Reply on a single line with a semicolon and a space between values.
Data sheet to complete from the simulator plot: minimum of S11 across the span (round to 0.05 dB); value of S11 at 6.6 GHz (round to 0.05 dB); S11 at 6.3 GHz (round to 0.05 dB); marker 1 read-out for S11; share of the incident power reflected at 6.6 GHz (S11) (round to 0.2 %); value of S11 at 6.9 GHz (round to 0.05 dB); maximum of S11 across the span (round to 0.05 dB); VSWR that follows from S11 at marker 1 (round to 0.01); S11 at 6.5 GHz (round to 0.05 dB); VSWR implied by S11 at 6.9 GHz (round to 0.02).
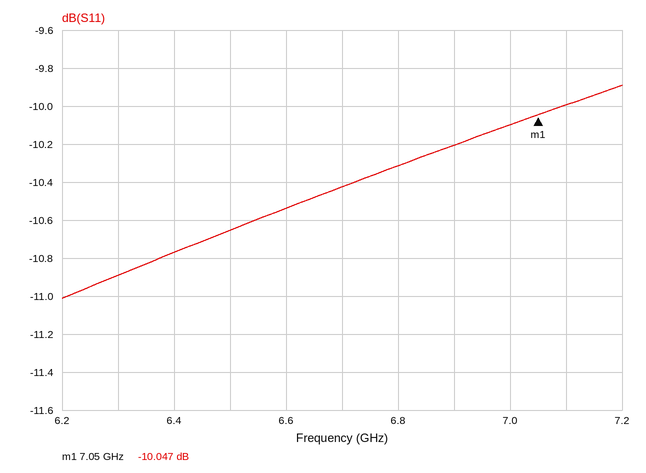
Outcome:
-11.00 dB; -10.55 dB; -10.90 dB; -10.047 dB; 8.8 %; -10.20 dB; -9.90 dB; 1.92; -10.65 dB; 1.90
